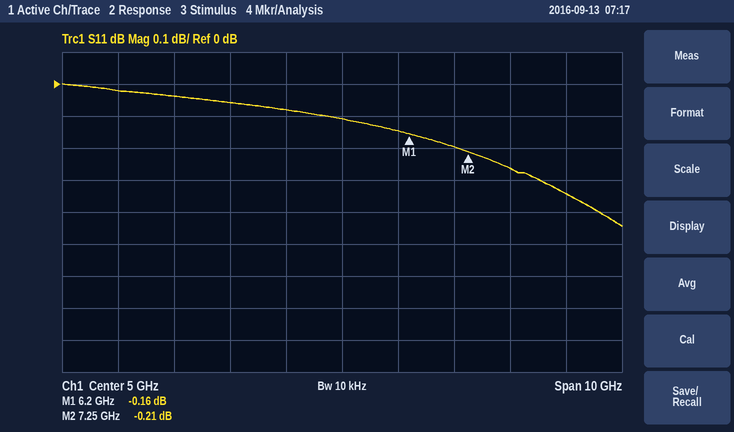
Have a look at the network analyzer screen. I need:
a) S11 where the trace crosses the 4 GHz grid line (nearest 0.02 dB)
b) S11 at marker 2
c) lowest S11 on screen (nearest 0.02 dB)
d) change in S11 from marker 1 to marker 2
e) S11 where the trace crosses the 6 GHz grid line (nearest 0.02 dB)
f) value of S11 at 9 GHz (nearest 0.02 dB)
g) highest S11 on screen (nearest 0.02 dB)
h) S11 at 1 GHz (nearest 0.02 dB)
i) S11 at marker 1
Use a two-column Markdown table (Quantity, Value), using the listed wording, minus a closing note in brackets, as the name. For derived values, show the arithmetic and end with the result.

| Quantity | Value |
|---|---|
| S11 where the trace crosses the 4 GHz grid line | -0.08 dB |
| S11 at marker 2 | -0.21 dB |
| lowest S11 on screen | -0.44 dB |
| change in S11 from marker 1 to marker 2 | -0.21 − (-0.16) = -0.05 dB |
| S11 where the trace crosses the 6 GHz grid line | -0.14 dB |
| value of S11 at 9 GHz | -0.34 dB |
| highest S11 on screen | 0.00 dB |
| S11 at 1 GHz | -0.02 dB |
| S11 at marker 1 | -0.16 dB |
